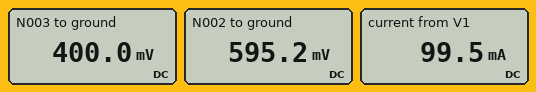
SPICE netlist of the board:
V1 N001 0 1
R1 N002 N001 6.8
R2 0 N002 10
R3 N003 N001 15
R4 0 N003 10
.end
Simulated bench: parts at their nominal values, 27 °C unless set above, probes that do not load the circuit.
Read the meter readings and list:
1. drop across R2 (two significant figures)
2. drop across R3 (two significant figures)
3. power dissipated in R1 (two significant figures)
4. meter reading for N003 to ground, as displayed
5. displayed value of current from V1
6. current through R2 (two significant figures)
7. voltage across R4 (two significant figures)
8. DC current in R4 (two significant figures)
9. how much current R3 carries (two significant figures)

600 mV
600 mV
24 mW
400.0 mV
99.5 mA
60 mA
400 mV
40 mA
40 mA
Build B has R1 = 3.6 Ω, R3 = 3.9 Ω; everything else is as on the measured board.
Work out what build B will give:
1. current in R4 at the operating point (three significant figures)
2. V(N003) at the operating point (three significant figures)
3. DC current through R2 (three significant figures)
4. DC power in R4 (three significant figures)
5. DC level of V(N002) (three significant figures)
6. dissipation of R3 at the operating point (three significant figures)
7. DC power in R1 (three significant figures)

71.9 mA
719 mV
73.5 mA
51.8 mW
735 mV
20.2 mW
19.5 mW
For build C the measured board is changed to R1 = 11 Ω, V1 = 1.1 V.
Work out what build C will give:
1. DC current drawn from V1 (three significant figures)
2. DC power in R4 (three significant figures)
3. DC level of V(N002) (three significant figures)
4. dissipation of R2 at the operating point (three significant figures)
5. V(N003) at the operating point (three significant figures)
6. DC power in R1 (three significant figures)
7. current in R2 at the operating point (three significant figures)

96.4 mA
19.4 mW
524 mV
27.4 mW
440 mV
30.2 mW
52.4 mA
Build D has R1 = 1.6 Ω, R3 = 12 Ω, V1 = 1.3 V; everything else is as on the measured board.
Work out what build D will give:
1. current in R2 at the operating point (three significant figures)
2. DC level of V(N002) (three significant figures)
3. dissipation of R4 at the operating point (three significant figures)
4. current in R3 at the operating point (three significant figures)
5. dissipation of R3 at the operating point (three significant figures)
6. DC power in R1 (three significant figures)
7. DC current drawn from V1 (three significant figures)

112 mA
1.12 V
34.9 mW
59.1 mA
41.9 mW
20.1 mW
171 mA
